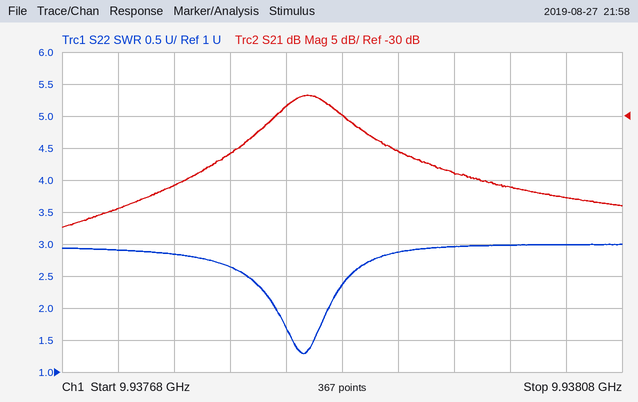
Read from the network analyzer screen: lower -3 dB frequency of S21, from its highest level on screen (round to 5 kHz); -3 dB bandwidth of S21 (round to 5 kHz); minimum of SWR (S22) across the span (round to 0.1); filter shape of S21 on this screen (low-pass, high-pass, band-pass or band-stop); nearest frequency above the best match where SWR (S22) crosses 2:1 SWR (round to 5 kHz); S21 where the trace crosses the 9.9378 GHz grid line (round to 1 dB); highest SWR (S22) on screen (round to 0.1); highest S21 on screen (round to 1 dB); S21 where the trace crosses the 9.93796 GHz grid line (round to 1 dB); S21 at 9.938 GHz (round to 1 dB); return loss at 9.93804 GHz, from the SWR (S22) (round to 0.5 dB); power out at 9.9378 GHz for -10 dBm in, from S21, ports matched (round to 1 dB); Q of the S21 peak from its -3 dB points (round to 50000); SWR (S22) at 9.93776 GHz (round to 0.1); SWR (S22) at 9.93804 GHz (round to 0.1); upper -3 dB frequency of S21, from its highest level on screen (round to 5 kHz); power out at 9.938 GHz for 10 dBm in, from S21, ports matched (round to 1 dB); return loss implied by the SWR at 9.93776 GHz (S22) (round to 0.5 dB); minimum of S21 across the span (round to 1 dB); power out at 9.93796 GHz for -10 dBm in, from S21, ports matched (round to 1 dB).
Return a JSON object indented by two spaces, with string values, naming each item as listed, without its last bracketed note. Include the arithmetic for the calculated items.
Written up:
{
  "lower -3 dB frequency of S21, from its highest level on screen": "9.937835 GHz",
  "-3 dB bandwidth of S21": "9.937880 GHz − 9.937835 GHz = 45 kHz",
  "minimum of SWR (S22) across the span": "1.3",
  "filter shape of S21 on this screen": "band-pass",
  "nearest frequency above the best match where SWR (S22) crosses 2:1 SWR": "9.937870 GHz",
  "S21 where the trace crosses the 9.9378 GHz grid line": "-36 dB",
  "highest SWR (S22) on screen": "3.0",
  "highest S21 on screen": "-27 dB",
  "S21 where the trace crosses the 9.93796 GHz grid line": "-39 dB",
  "S21 at 9.938 GHz": "-41 dB",
  "return loss at 9.93804 GHz, from the SWR (S22)": "−20 log10((3 − 1)/(3 + 1)) ≈ 6.0 dB",
  "power out at 9.9378 GHz for -10 dBm in, from S21, ports matched": "-10 dBm + (-36 dB) = -46 dBm",
  "Q of the S21 peak from its -3 dB points": "9.93786 GHz / 45 kHz ≈ 220841, so 200000 to the nearest 50000",
  "SWR (S22) at 9.93776 GHz": "2.8",
  "SWR (S22) at 9.93804 GHz": "3.0",
  "upper -3 dB frequency of S21, from its highest level on screen": "9.937880 GHz",
  "power out at 9.938 GHz for 10 dBm in, from S21, ports matched": "10 dBm + (-41 dB) = -31 dBm",
  "return loss implied by the SWR at 9.93776 GHz (S22)": "−20 log10((2.8 − 1)/(2.8 + 1)) ≈ 6.5 dB",
  "minimum of S21 across the span": "-47 dB",
  "power out at 9.93796 GHz for -10 dBm in, from S21, ports matched": "-10 dBm + (-39 dB) = -49 dBm"
}
